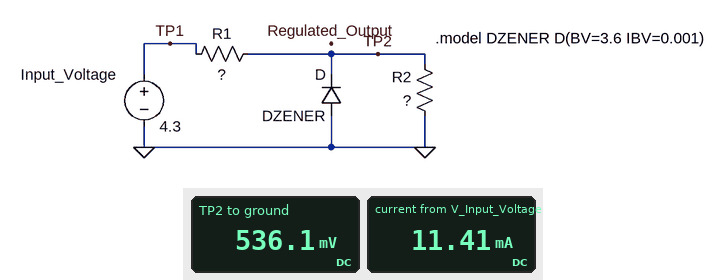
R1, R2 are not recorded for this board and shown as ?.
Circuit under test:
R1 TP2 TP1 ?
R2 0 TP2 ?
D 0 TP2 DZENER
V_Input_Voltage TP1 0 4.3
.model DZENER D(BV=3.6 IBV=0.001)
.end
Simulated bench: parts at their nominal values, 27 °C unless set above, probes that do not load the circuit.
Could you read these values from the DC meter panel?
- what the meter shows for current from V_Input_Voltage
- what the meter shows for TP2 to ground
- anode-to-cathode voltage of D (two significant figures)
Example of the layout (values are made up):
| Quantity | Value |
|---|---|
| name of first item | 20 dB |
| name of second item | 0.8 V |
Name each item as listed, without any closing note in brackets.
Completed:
| Quantity | Value |
|---|---|
| what the meter shows for current from V_Input_Voltage | 11.41 mA |
| what the meter shows for TP2 to ground | 536.1 mV |
| anode-to-cathode voltage of D | -540 mV |
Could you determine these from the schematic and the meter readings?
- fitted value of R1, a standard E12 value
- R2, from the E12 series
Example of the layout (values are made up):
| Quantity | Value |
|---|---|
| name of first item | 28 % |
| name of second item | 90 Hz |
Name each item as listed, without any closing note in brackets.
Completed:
| Quantity | Value |
|---|---|
| fitted value of R1, a standard E12 value | 330 Ω |
| R2, from the E12 series | 47 Ω |
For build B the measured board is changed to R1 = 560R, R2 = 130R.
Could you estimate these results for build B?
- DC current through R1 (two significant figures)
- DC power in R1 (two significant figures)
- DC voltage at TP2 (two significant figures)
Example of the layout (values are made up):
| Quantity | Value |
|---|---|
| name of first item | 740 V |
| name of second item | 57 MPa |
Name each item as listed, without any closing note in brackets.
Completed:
| Quantity | Value |
|---|---|
| DC current through R1 | 6.2 mA |
| DC power in R1 | 22 mW |
| DC voltage at TP2 | 810 mV |
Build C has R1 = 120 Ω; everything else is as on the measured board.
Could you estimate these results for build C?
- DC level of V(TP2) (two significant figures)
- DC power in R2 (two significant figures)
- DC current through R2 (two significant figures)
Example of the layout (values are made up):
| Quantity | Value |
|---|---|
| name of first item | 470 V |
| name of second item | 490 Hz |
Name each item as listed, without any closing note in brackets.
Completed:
| Quantity | Value |
|---|---|
| DC level of V(TP2) | 1.2 V |
| DC power in R2 | 31 mW |
| DC current through R2 | 26 mA |
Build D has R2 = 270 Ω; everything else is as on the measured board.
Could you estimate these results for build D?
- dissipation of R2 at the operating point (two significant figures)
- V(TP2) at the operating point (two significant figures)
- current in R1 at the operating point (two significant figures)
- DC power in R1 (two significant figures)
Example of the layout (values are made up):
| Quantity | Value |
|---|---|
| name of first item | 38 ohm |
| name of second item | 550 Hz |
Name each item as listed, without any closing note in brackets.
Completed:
| Quantity | Value |
|---|---|
| dissipation of R2 at the operating point | 14 mW |
| V(TP2) at the operating point | 1.9 V |
| current in R1 at the operating point | 7.2 mA |
| DC power in R1 | 17 mW |
